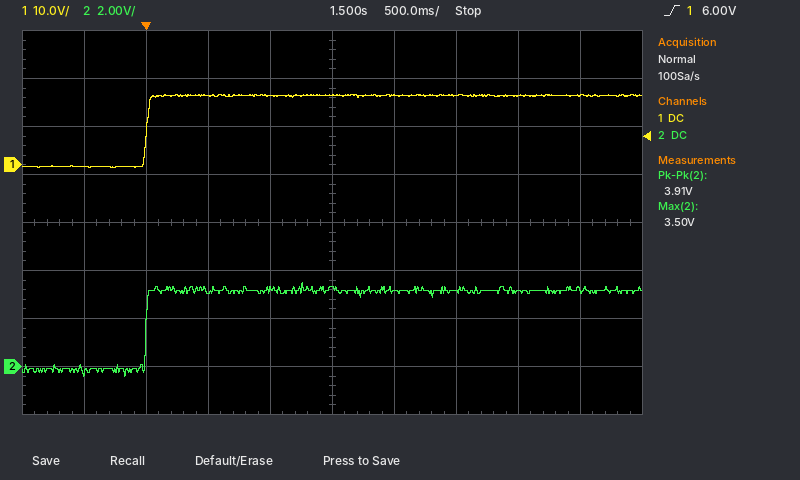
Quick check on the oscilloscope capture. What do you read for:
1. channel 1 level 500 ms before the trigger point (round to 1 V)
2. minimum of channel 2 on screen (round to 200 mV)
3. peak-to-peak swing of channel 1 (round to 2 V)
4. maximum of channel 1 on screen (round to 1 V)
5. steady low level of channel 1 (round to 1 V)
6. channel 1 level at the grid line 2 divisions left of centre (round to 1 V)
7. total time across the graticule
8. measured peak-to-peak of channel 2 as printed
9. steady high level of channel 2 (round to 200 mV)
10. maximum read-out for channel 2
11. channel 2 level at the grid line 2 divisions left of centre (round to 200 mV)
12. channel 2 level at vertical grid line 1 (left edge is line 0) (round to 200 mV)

0 V
-400 mV
16 V
15 V
0 V
14 V
5 s
3.91 V
3.2 V
3.50 V
3.2 V
-200 mV
